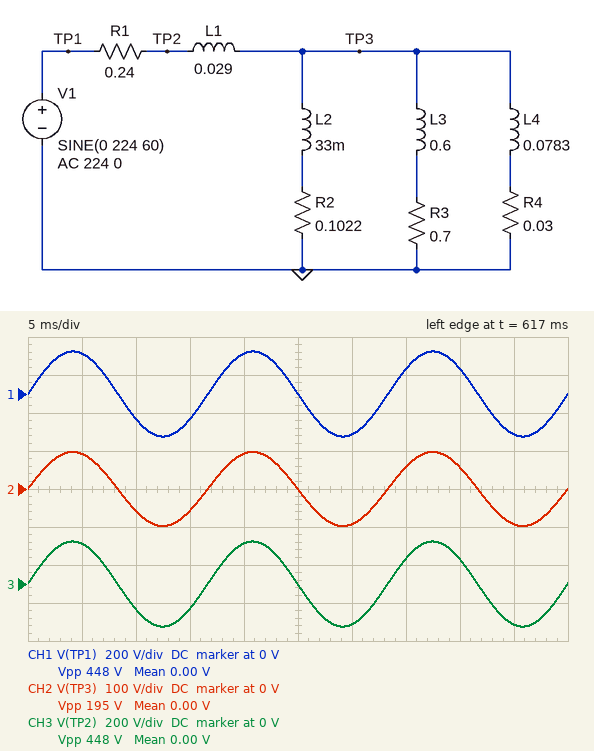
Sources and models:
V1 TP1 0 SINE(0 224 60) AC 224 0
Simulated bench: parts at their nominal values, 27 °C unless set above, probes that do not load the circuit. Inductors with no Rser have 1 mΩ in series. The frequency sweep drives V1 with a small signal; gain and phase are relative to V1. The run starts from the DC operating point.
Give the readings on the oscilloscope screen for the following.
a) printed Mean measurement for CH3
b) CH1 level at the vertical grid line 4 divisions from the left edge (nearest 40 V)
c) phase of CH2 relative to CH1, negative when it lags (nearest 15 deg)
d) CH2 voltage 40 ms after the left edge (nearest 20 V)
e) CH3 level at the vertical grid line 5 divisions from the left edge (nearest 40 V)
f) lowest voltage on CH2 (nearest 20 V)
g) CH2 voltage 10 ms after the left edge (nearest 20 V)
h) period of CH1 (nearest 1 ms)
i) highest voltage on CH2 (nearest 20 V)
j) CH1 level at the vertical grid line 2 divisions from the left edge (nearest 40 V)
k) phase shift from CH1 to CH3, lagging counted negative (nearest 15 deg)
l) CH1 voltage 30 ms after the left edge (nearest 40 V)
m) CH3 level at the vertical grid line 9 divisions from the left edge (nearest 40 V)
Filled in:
0.00 V
200 V
0 deg
60 V
0 V
-100 V
-60 V
17 ms
100 V
-120 V
0 deg
-200 V
-200 V
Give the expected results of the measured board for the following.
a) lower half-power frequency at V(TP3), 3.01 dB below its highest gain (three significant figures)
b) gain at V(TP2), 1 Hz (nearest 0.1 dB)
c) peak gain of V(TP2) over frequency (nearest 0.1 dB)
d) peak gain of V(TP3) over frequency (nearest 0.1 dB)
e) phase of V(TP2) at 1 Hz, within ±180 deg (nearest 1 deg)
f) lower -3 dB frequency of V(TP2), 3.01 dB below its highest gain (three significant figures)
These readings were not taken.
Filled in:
670 mHz
-2.4 dB
0 dB
-7.2 dB
33 deg
854 mHz
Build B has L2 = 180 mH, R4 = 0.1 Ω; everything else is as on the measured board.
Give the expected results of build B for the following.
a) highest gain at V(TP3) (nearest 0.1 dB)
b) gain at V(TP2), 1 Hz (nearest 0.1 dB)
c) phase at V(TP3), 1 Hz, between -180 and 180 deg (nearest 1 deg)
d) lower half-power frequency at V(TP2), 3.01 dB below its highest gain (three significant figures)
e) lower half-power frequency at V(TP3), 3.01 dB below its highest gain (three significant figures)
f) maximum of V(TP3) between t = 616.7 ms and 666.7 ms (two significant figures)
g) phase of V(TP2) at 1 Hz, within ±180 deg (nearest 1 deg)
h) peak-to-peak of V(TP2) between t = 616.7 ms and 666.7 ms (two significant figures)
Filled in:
-4.0 dB
-1.3 dB
21 deg
570 mHz
536 mHz
140 V
24 deg
450 V
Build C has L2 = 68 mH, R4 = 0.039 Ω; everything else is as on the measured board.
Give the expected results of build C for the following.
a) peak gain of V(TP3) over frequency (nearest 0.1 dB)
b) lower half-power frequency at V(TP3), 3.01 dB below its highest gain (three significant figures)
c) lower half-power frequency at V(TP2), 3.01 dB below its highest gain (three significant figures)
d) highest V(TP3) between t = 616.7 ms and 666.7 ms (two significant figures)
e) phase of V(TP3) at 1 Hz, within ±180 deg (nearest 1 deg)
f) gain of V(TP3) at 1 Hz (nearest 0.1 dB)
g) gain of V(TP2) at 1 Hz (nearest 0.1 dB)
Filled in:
-5.3 dB
642 mHz
679 mHz
120 V
25 deg
-6.9 dB
-1.7 dB
